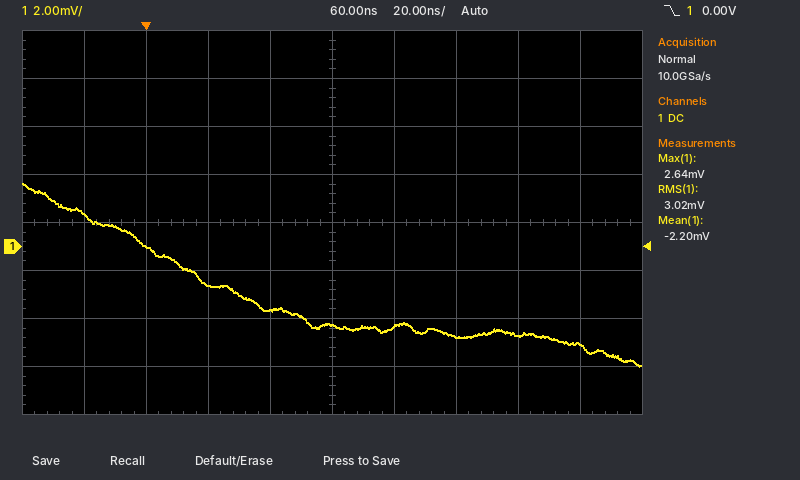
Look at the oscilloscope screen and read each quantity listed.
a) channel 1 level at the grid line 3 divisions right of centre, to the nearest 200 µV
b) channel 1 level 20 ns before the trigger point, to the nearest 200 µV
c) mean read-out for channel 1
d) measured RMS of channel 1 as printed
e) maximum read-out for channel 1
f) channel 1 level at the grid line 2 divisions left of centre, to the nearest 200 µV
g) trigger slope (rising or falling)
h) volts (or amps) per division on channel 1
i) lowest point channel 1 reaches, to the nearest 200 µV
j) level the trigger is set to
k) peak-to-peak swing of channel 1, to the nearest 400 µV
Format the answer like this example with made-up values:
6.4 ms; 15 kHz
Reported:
-3.8 mV; 1.4 mV; -2.20 mV; 3.02 mV; 2.64 mV; -1.6 mV; falling; 2 mV; -5.0 mV; 0.00 V; 7.6 mV
